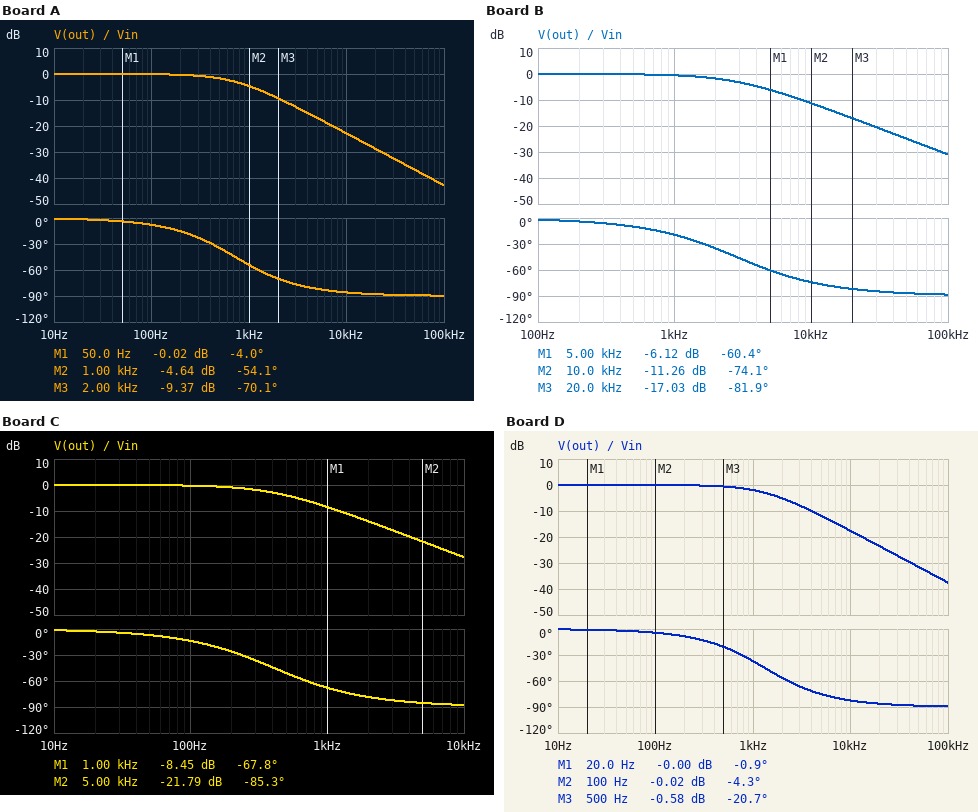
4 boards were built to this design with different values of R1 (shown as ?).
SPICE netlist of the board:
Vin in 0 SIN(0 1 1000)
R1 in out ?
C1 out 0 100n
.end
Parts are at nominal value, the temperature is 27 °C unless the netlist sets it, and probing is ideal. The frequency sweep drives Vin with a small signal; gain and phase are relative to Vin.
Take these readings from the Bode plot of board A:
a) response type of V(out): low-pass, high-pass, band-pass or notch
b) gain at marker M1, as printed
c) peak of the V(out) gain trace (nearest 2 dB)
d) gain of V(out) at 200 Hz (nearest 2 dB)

low-pass
-0.02 dB
0 dB
0 dB
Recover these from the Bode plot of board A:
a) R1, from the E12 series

2.2 kΩ
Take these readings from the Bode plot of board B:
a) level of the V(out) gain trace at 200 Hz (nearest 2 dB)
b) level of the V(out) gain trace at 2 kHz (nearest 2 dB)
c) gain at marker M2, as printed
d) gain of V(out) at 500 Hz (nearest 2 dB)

0 dB
-2 dB
-11.26 dB
0 dB
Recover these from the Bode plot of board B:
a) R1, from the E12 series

560 Ω
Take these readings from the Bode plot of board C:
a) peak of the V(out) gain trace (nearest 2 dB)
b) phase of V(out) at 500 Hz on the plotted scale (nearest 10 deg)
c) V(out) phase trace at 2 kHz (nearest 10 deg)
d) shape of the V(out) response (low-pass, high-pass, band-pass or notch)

0 dB
-50 deg
-80 deg
low-pass
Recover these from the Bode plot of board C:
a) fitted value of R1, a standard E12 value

3.9 kΩ
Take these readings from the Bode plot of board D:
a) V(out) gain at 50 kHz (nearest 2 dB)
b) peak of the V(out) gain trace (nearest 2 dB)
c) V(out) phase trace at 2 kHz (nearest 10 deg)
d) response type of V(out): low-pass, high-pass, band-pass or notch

-32 dB
0 dB
-60 deg
low-pass
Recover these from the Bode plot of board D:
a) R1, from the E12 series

1.2 kΩ
